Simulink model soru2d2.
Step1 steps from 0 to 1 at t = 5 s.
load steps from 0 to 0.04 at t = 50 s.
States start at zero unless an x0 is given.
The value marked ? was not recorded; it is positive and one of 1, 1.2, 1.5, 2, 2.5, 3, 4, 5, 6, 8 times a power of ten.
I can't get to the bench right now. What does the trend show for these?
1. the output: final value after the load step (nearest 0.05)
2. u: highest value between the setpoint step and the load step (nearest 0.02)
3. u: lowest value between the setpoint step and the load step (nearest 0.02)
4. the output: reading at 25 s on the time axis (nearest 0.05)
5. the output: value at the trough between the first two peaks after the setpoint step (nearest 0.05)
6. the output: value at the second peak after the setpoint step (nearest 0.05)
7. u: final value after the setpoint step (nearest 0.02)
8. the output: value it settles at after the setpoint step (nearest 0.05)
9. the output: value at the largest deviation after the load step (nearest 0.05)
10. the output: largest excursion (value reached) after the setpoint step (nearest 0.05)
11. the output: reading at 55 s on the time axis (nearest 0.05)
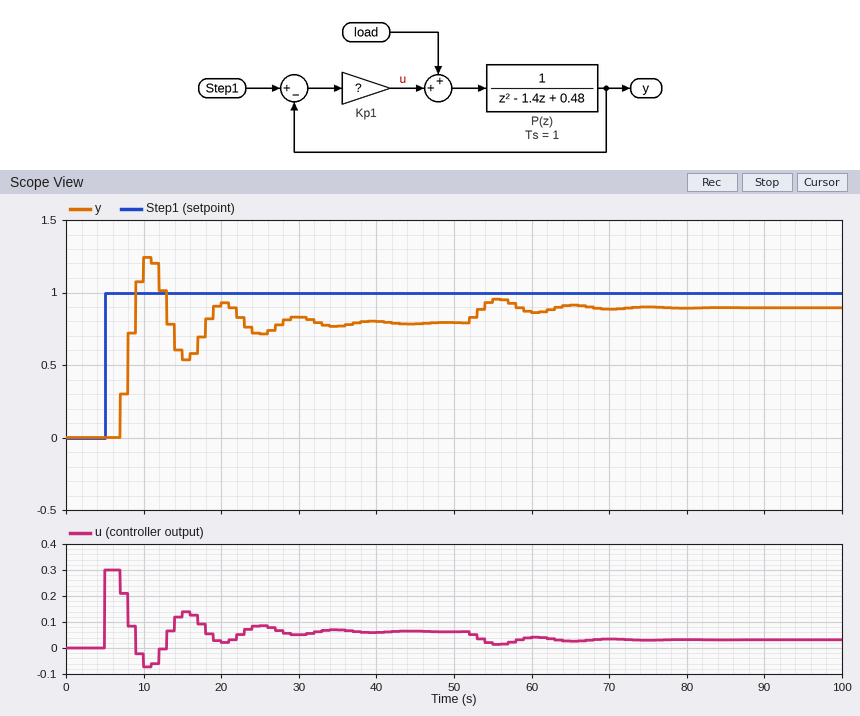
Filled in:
0.90
0.30
-0.08
0.70
0.55
0.95
0.06
0.80
0.95
1.25
0.95
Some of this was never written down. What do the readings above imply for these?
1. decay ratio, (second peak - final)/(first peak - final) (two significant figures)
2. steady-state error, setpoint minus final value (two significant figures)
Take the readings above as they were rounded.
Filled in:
0.33
0.20
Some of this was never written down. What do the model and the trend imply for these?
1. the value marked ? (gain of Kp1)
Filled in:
0.3
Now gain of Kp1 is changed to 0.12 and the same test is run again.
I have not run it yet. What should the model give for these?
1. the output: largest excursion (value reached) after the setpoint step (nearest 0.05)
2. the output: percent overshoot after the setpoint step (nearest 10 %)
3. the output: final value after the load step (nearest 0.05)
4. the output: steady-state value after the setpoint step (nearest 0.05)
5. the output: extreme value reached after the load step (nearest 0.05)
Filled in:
0.70
20 %
0.80
0.60
0.85
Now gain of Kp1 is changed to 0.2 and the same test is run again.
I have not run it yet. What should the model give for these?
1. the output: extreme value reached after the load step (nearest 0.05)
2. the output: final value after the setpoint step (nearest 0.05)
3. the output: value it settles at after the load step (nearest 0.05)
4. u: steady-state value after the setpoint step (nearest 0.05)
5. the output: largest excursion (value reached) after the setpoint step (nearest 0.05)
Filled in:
0.90
0.70
0.85
0.05
0.95
